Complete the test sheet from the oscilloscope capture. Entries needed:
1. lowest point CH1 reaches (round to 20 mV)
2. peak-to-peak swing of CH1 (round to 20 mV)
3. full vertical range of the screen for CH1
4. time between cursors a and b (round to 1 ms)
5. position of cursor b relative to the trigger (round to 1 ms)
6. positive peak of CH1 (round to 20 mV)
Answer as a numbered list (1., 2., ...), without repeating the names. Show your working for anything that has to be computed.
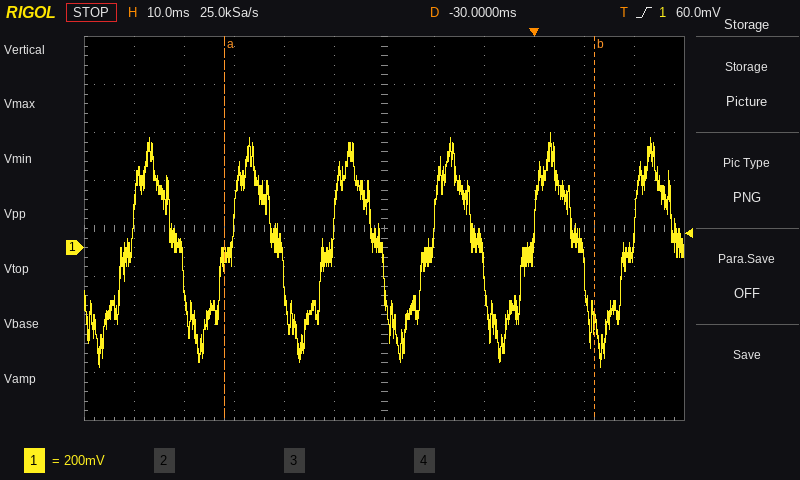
1. -500 mV
2. 480 mV − (-500 mV) = 980 mV
3. 1.6 V
4. 74 ms
5. +12 ms
6. 480 mV
